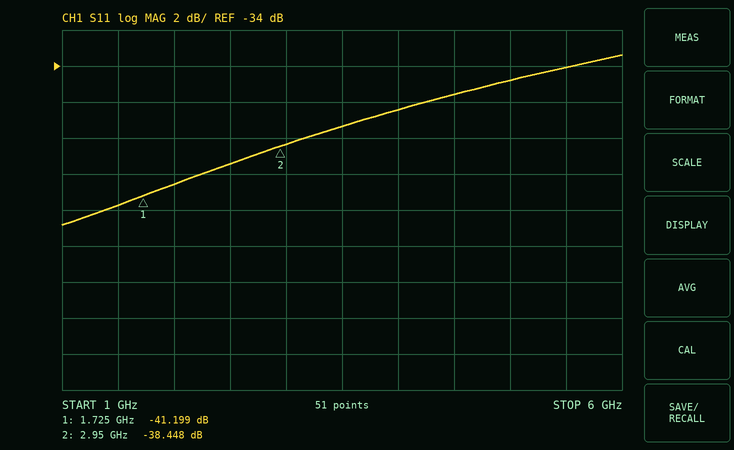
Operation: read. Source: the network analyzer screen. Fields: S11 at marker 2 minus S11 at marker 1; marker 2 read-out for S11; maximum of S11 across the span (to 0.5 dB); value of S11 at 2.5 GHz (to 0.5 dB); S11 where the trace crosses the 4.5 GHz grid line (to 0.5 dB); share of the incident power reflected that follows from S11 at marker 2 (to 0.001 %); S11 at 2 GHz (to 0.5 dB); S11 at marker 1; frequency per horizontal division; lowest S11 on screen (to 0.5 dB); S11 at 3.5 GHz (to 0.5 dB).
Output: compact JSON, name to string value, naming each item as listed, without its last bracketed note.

{"S11 at marker 2 minus S11 at marker 1": "2.751 dB", "marker 2 read-out for S11": "-38.448 dB", "maximum of S11 across the span": "-33.5 dB", "value of S11 at 2.5 GHz": "-39.5 dB", "S11 where the trace crosses the 4.5 GHz grid line": "-35.5 dB", "share of the incident power reflected that follows from S11 at marker 2": "0.014 %", "S11 at 2 GHz": "-40.5 dB", "S11 at marker 1": "-41.199 dB", "frequency per horizontal division": "500 MHz", "lowest S11 on screen": "-43.0 dB", "S11 at 3.5 GHz": "-37.5 dB"}
